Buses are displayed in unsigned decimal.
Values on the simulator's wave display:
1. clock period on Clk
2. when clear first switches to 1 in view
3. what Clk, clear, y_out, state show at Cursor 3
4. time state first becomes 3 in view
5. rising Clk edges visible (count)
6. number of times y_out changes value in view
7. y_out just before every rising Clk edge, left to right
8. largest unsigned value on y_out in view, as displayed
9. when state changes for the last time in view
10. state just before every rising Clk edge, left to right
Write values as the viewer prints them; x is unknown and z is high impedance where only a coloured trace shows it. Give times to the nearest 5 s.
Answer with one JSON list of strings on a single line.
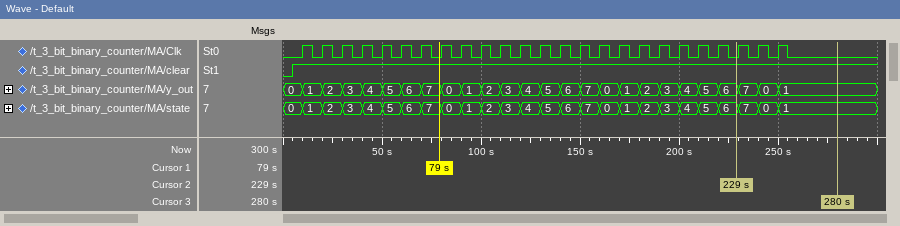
["10 s", "5 s", "Clk=0, clear=1, y_out=1, state=1", "30 s", "25", "25", "0, 1, 2, 3, 4, 5, 6, 7, 0, 1, 2, 3, 4, 5, 6, 7, 0, 1, 2, 3, 4, 5, 6, 7, 0", "7", "250 s", "0, 1, 2, 3, 4, 5, 6, 7, 0, 1, 2, 3, 4, 5, 6, 7, 0, 1, 2, 3, 4, 5, 6, 7, 0"]
